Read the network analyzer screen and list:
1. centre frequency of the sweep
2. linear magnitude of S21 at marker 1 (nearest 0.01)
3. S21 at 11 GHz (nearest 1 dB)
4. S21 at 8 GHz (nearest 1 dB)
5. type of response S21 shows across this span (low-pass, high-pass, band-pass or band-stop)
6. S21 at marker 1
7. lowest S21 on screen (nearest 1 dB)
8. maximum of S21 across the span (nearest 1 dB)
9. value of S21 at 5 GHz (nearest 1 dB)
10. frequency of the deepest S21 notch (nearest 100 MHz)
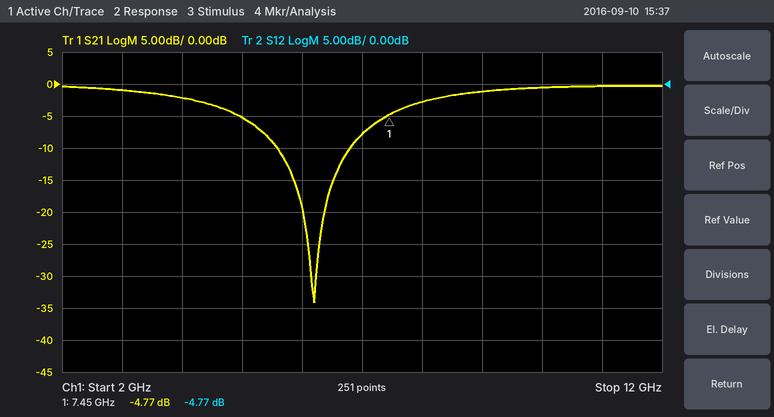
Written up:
7 GHz
0.58
0 dB
-3 dB
band-stop
-4.77 dB
-34 dB
0 dB
-5 dB
6.2 GHz
